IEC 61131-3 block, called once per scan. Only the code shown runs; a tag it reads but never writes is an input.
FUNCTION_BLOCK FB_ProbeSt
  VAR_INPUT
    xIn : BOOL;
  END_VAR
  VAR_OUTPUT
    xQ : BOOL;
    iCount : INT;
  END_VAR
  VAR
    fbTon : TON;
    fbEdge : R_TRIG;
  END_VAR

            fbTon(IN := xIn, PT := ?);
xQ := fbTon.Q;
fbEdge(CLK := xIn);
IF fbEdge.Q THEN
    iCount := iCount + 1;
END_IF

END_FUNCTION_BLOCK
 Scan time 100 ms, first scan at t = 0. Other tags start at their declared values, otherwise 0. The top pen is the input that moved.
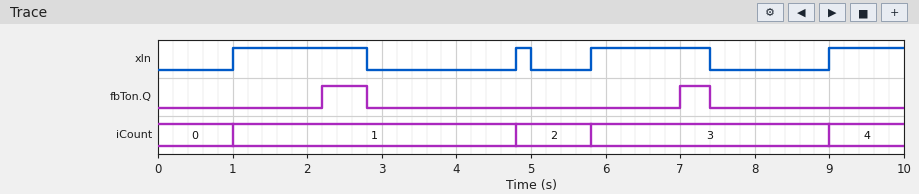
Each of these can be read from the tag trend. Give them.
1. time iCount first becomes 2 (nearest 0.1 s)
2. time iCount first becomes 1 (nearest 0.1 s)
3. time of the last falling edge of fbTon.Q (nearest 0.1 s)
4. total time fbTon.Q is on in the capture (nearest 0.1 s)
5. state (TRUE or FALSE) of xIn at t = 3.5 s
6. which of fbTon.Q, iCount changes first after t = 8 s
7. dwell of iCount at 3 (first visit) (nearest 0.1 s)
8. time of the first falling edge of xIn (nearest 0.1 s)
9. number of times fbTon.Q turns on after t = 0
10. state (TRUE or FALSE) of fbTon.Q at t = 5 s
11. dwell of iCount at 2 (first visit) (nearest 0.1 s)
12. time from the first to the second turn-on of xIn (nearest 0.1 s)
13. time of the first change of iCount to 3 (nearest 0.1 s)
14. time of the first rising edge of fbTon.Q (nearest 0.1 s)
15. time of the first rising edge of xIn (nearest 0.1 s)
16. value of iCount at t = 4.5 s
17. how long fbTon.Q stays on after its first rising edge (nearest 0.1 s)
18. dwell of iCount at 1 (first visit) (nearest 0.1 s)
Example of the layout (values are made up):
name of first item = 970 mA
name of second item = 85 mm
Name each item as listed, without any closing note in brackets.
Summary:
time iCount first becomes 2 = 4.8 s
time iCount first becomes 1 = 1.0 s
time of the last falling edge of fbTon.Q = 7.4 s
total time fbTon.Q is on in the capture = 1.0 s
state (TRUE or FALSE) of xIn at t = 3.5 s = FALSE
which of fbTon.Q, iCount changes first after t = 8 s = iCount
dwell of iCount at 3 (first visit) = 3.2 s
time of the first falling edge of xIn = 2.8 s
number of times fbTon.Q turns on after t = 0 = 2
state (TRUE or FALSE) of fbTon.Q at t = 5 s = FALSE
dwell of iCount at 2 (first visit) = 1.0 s
time from the first to the second turn-on of xIn = 3.8 s
time of the first change of iCount to 3 = 5.8 s
time of the first rising edge of fbTon.Q = 2.2 s
time of the first rising edge of xIn = 1.0 s
value of iCount at t = 4.5 s = 1
how long fbTon.Q stays on after its first rising edge = 0.6 s
dwell of iCount at 1 (first visit) = 3.8 s
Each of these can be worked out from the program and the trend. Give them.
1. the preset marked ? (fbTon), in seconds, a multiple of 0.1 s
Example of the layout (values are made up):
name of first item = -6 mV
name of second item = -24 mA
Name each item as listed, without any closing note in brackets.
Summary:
the preset marked ? (fbTon), in seconds, a multiple of 0.1 s = 1.2 s
